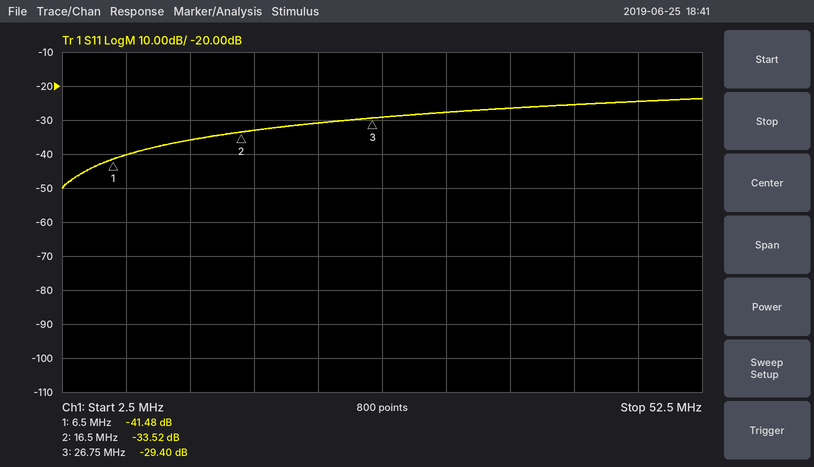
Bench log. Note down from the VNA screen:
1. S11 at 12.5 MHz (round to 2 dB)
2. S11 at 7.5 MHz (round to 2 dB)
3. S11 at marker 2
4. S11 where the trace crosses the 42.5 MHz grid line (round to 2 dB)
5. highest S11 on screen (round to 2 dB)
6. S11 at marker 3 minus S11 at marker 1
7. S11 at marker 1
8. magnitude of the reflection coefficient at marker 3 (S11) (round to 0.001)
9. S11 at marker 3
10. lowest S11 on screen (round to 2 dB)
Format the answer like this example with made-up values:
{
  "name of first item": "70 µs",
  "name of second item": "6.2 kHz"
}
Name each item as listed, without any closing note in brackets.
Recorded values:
{
  "S11 at 12.5 MHz": "-36 dB",
  "S11 at 7.5 MHz": "-40 dB",
  "S11 at marker 2": "-33.52 dB",
  "S11 where the trace crosses the 42.5 MHz grid line": "-26 dB",
  "highest S11 on screen": "-24 dB",
  "S11 at marker 3 minus S11 at marker 1": "12.08 dB",
  "S11 at marker 1": "-41.48 dB",
  "magnitude of the reflection coefficient at marker 3 (S11)": "0.034",
  "S11 at marker 3": "-29.40 dB",
  "lowest S11 on screen": "-50 dB"
}
